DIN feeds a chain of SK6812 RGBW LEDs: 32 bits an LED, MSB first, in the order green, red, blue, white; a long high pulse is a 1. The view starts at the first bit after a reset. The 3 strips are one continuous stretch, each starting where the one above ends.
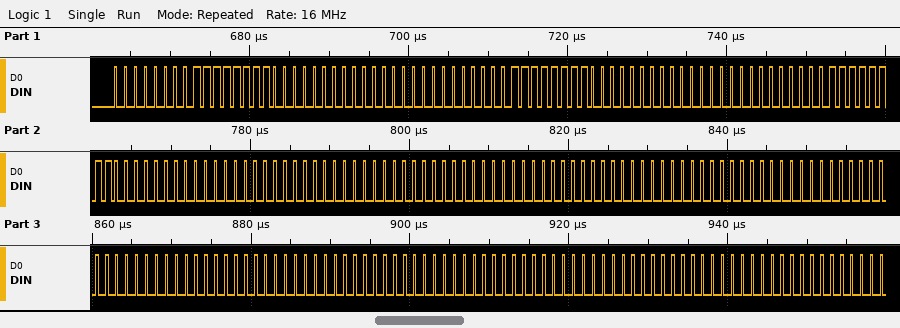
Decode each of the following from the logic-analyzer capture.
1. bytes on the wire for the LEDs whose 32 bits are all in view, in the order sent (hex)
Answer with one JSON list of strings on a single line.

["00 FF 00 00 00 FF 00 00 00 FF 00 00 00 00 00 00 00 00 00 00 00 00 00 00 00 00 00 00"]
